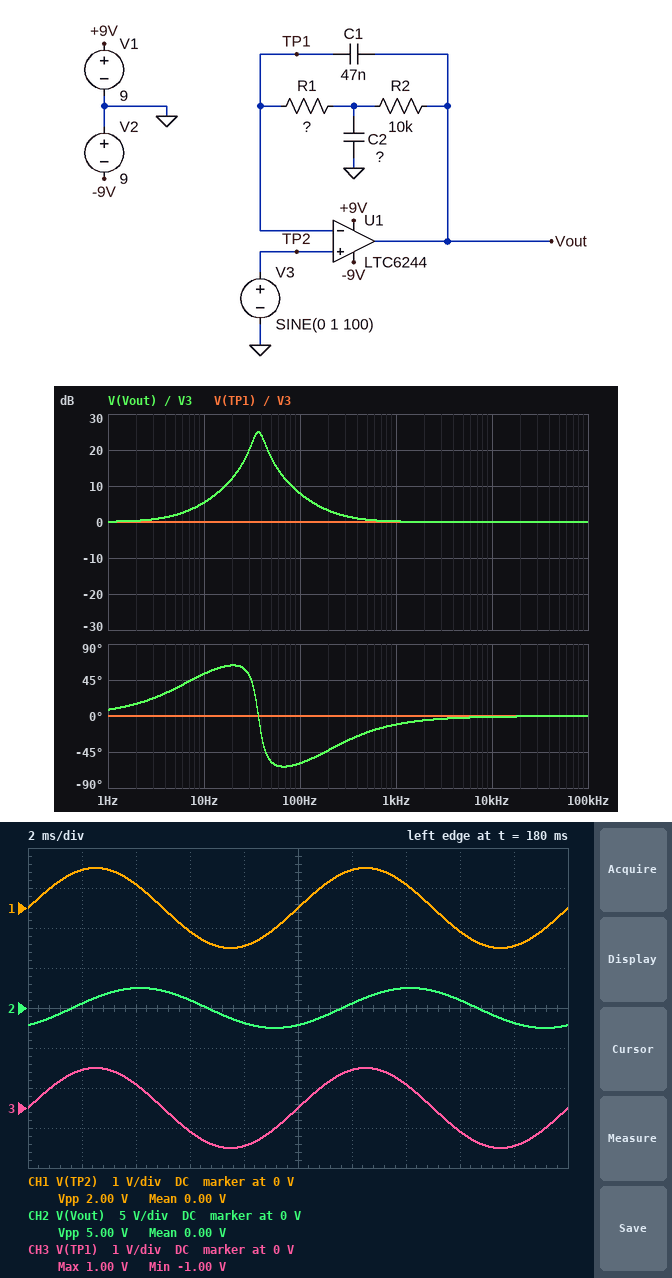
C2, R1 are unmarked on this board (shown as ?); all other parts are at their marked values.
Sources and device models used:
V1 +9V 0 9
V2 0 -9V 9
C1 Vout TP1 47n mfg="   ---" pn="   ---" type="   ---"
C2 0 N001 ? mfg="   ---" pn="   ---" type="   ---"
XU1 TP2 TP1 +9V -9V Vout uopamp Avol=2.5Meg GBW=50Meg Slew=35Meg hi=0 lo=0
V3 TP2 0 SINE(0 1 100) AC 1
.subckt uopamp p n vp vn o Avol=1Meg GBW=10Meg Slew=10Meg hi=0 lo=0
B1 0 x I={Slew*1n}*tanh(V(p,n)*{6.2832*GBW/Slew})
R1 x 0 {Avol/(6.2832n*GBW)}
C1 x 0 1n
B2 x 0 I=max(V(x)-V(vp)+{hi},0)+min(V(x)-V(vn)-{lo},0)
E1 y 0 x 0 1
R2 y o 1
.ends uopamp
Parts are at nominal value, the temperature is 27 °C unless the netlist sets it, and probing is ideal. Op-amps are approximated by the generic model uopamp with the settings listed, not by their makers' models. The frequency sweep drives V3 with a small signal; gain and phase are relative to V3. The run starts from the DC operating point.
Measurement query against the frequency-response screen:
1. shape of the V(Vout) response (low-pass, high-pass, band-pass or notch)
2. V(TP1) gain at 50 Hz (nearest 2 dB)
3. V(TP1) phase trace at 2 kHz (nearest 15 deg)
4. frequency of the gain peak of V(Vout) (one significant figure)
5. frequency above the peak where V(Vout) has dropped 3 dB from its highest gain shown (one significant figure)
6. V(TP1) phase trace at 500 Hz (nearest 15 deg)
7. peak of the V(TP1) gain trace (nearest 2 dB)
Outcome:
band-pass
0 dB
0 deg
40 Hz
40 Hz
0 deg
0 dB
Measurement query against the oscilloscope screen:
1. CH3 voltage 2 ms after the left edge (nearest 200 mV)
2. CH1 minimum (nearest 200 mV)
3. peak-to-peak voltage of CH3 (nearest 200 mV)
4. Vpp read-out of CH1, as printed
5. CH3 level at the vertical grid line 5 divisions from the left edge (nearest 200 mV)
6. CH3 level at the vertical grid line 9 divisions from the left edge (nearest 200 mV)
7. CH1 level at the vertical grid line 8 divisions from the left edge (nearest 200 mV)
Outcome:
1.0 V
-1.0 V
2.0 V
2.00 V
0 V
-1.0 V
-600 mV
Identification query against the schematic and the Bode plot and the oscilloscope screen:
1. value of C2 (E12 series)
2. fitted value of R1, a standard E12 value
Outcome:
2.2 µF
18 kΩ
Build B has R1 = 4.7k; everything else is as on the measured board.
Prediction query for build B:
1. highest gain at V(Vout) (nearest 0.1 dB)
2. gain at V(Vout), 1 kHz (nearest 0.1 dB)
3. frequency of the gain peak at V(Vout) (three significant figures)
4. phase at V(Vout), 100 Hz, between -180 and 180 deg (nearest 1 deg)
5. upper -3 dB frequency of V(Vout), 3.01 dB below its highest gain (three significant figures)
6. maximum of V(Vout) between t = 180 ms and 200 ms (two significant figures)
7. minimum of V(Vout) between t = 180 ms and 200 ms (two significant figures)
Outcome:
30.3 dB
1.9 dB
72.2 Hz
-61 deg
84.4 Hz
9.0 V
-9.0 V
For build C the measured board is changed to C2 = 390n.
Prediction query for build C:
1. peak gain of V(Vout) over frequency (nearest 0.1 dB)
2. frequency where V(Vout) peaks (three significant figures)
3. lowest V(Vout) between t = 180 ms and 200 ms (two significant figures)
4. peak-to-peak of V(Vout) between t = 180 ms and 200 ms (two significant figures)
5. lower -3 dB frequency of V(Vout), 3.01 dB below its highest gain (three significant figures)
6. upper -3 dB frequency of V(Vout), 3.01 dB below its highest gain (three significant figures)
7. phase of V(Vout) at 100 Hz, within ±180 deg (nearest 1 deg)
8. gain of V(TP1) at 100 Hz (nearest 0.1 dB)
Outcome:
12.0 dB
87.6 Hz
-3.7 V
7.5 V
60.0 Hz
128 Hz
-15 deg
0 dB
